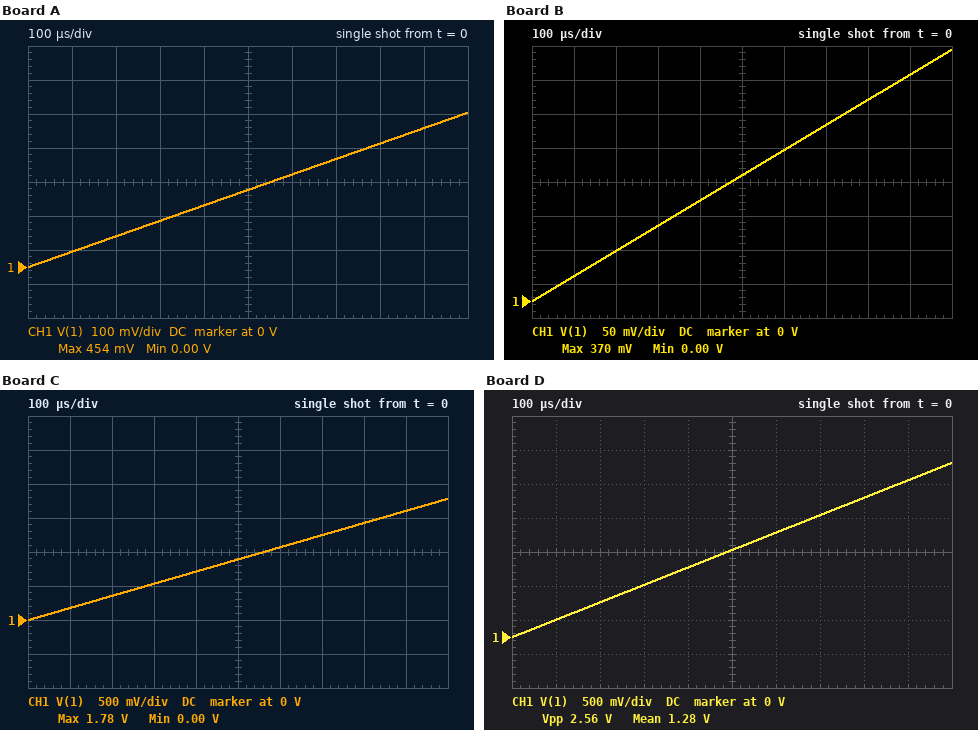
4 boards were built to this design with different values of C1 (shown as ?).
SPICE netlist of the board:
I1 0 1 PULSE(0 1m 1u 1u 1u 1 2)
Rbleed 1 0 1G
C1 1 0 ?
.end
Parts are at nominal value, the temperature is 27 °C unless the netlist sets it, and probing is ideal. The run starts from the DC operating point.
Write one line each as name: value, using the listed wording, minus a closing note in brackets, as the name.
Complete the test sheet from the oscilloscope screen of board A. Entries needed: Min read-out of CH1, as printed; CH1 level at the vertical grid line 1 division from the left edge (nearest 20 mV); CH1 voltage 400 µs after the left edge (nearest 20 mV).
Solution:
Min read-out of CH1, as printed: 0.00 V
CH1 level at the vertical grid line 1 division from the left edge: 40 mV
CH1 voltage 400 µs after the left edge: 180 mV
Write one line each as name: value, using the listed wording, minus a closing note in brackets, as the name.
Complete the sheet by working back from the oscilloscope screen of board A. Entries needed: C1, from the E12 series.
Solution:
C1, from the E12 series: 2.2 µF
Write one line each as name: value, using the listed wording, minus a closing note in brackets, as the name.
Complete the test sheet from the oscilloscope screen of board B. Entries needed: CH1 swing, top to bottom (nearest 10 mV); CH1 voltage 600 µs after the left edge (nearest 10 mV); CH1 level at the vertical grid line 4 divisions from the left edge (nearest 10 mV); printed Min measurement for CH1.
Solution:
CH1 swing, top to bottom: 370 mV
CH1 voltage 600 µs after the left edge: 220 mV
CH1 level at the vertical grid line 4 divisions from the left edge: 150 mV
printed Min measurement for CH1: 0.00 V
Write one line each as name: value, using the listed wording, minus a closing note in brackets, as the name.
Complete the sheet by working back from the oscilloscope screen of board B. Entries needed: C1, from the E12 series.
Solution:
C1, from the E12 series: 2.7 µF
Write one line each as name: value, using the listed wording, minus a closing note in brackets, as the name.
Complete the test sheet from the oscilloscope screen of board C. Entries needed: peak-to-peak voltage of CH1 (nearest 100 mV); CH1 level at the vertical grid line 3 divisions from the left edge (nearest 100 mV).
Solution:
peak-to-peak voltage of CH1: 1.8 V
CH1 level at the vertical grid line 3 divisions from the left edge: 500 mV
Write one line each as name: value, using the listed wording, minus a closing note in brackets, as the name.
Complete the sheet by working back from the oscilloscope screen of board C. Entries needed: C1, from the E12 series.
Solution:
C1, from the E12 series: 560 nF
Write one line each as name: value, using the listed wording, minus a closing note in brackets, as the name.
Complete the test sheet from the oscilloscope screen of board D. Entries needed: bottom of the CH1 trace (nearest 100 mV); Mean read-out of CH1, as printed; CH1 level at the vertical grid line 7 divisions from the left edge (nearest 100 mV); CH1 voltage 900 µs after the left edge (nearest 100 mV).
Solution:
bottom of the CH1 trace: 0 V
Mean read-out of CH1, as printed: 1.28 V
CH1 level at the vertical grid line 7 divisions from the left edge: 1.8 V
CH1 voltage 900 µs after the left edge: 2.3 V
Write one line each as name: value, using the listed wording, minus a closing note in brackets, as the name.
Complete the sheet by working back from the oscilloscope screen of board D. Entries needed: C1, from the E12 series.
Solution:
C1, from the E12 series: 390 nF
